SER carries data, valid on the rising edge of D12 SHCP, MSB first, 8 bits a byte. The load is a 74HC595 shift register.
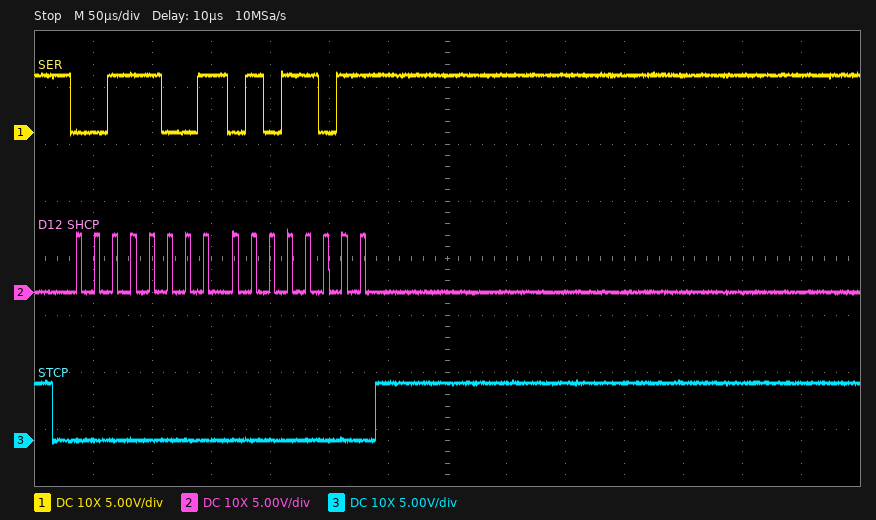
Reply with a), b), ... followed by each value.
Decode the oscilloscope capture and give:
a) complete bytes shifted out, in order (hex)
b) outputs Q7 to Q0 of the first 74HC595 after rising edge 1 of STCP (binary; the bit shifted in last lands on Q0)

a) 39 5B
b) 01011011
